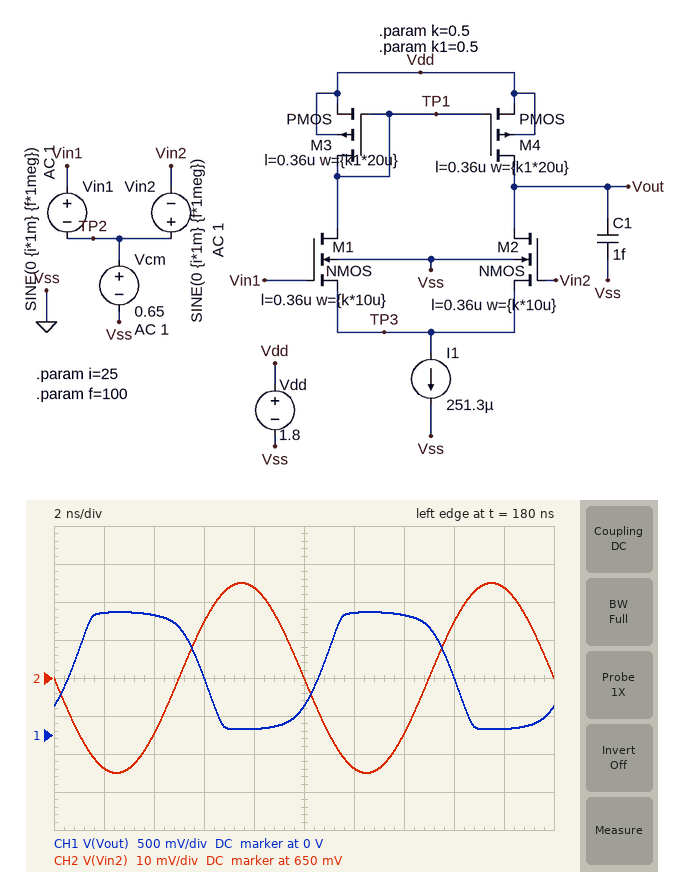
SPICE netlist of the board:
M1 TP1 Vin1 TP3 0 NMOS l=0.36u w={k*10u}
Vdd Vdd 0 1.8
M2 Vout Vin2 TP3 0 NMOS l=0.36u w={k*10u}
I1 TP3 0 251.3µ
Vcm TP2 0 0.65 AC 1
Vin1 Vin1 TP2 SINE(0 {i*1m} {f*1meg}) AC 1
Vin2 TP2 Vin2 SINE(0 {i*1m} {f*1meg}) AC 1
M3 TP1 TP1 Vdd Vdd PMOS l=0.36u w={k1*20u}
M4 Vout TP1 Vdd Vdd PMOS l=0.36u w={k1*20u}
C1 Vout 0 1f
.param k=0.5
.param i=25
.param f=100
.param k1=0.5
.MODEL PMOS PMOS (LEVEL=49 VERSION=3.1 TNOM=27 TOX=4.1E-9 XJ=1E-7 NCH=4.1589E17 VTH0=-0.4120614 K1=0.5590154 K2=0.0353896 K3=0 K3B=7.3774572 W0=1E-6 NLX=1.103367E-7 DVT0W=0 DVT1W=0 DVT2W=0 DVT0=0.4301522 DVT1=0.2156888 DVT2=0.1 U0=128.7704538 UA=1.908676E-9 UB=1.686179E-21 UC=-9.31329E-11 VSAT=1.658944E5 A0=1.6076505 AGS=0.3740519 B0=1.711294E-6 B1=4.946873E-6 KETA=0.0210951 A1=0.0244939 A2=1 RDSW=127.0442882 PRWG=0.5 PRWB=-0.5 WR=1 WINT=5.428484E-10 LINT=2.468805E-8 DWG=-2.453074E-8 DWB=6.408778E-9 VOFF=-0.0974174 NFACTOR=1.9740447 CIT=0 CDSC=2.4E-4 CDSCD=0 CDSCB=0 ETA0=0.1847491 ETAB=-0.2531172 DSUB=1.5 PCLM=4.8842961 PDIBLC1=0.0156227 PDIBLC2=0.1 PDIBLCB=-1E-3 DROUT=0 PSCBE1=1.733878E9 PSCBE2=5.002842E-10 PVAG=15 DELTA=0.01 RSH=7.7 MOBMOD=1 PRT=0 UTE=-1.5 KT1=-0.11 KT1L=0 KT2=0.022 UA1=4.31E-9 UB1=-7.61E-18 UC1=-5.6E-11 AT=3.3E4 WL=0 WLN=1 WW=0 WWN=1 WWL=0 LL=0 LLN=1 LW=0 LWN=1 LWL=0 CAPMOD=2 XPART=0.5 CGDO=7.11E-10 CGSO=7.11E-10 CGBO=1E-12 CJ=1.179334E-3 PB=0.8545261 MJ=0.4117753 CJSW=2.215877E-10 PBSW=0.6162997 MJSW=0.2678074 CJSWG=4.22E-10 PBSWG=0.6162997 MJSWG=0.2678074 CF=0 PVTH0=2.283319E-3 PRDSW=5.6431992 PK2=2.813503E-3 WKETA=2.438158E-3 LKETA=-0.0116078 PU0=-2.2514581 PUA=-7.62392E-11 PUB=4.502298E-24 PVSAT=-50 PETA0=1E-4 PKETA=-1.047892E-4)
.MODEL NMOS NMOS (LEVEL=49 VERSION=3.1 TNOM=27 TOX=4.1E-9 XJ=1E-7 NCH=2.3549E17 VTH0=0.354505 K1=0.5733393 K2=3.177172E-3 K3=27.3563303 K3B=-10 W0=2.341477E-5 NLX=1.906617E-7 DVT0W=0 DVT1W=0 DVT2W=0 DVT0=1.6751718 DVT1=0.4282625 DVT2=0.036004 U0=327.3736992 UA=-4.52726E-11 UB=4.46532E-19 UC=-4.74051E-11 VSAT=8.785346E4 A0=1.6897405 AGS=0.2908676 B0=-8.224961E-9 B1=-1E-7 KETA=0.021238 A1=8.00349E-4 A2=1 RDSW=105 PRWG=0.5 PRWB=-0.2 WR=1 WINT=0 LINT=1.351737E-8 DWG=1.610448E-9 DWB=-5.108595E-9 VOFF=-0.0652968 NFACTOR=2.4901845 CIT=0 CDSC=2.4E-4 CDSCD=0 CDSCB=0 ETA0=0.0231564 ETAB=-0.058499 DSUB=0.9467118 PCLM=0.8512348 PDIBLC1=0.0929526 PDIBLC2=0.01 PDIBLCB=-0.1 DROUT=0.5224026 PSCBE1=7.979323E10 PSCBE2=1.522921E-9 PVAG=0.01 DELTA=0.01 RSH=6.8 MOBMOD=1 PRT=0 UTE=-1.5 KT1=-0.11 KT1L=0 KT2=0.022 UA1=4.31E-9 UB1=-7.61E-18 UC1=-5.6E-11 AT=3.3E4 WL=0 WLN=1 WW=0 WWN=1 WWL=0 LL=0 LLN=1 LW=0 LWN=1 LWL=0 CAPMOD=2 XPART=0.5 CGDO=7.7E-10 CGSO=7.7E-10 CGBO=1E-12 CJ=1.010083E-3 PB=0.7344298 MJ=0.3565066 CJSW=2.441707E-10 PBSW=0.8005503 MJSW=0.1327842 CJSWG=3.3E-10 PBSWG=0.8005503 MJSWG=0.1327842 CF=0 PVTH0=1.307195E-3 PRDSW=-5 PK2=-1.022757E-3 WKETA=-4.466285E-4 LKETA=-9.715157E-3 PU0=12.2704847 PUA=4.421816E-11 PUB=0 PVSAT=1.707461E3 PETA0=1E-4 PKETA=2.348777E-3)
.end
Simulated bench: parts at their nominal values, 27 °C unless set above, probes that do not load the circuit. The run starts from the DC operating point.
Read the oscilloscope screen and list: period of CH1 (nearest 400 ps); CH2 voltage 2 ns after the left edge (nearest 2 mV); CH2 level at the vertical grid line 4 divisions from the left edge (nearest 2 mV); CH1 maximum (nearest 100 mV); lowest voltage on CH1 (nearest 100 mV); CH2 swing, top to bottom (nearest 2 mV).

10.0 ns
626 mV
674 mV
1.6 V
100 mV
50 mV
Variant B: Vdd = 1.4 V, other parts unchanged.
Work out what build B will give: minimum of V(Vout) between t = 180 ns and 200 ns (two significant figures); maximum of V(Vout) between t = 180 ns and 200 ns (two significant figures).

55 mV
1.2 V
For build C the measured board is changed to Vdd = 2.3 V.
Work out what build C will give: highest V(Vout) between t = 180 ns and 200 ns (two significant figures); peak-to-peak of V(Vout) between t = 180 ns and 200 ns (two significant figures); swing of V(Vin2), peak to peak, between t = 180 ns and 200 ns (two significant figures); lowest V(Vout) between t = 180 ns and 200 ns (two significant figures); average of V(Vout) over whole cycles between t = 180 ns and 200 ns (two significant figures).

2.1 V
2.0 V
50 mV
100 mV
1.2 V
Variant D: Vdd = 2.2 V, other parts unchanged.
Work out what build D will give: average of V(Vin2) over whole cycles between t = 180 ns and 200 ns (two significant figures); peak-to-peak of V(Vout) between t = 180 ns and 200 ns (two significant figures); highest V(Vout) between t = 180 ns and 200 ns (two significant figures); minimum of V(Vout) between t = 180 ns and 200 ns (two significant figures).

650 mV
1.9 V
2.0 V
96 mV
